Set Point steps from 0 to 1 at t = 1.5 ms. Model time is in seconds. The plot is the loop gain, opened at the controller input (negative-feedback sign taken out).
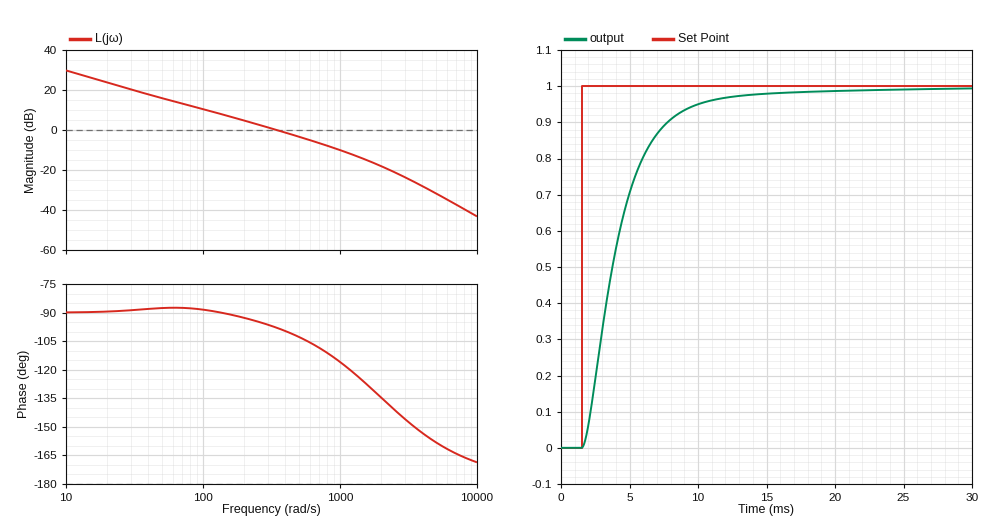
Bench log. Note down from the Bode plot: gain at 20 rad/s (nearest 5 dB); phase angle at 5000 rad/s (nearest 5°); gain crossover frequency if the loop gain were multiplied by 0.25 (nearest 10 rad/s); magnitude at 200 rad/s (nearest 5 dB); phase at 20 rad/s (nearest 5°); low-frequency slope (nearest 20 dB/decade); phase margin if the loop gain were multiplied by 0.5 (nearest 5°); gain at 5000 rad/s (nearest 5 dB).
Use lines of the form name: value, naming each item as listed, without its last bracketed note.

gain at 20 rad/s: 25 dB
phase angle at 5000 rad/s: -160°
gain crossover frequency if the loop gain were multiplied by 0.25: 80 rad/s
magnitude at 200 rad/s: 5 dB
phase at 20 rad/s: -90°
low-frequency slope: -20 dB/decade
phase margin if the loop gain were multiplied by 0.5: 90°
gain at 5000 rad/s: -30 dB
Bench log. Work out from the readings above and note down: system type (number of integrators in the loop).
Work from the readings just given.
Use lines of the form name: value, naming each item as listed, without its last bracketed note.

system type: 1
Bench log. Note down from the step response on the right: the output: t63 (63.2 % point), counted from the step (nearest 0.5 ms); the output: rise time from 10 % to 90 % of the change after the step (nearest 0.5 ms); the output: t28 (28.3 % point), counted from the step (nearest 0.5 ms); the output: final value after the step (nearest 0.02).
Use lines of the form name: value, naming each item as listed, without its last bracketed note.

the output: t63 (63.2 % point), counted from the step: 3.0 ms
the output: rise time from 10 % to 90 % of the change after the step: 5.5 ms
the output: t28 (28.3 % point), counted from the step: 1.5 ms
the output: final value after the step: 1.00
